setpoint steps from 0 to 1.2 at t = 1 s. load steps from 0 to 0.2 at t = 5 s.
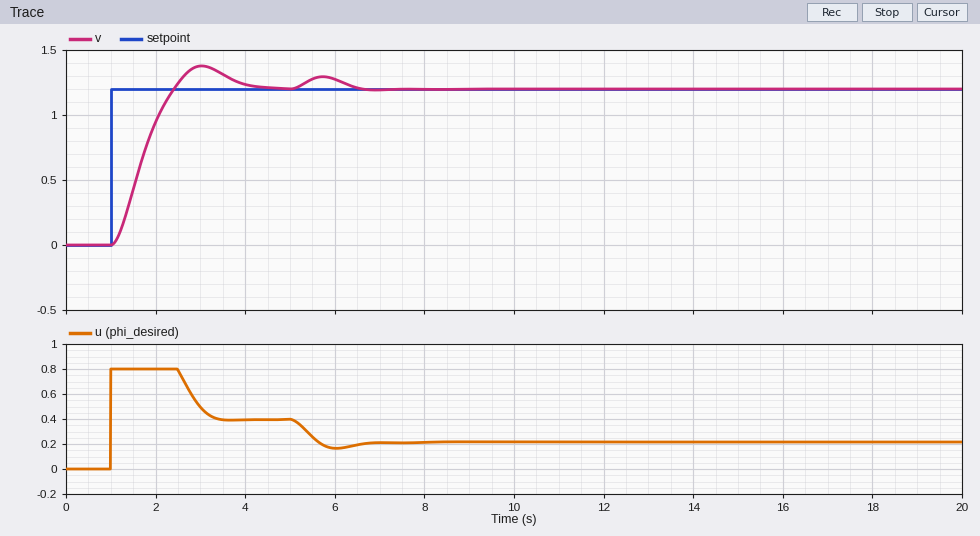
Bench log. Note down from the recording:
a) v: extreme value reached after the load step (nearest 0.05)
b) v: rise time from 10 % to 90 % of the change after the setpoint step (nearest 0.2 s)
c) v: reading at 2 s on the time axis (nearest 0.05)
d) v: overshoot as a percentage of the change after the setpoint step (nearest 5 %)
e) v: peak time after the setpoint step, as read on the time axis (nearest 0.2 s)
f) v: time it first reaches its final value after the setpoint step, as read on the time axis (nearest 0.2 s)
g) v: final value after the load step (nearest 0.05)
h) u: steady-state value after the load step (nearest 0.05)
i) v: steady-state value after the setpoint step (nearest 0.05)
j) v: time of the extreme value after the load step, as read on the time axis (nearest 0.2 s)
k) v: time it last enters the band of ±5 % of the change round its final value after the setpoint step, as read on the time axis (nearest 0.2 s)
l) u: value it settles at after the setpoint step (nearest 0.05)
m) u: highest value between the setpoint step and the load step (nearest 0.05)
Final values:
1.30
1.0 s
0.95
15 %
3.0 s
2.4 s
1.20
0.20
1.20
5.8 s
3.8 s
0.40
0.80
